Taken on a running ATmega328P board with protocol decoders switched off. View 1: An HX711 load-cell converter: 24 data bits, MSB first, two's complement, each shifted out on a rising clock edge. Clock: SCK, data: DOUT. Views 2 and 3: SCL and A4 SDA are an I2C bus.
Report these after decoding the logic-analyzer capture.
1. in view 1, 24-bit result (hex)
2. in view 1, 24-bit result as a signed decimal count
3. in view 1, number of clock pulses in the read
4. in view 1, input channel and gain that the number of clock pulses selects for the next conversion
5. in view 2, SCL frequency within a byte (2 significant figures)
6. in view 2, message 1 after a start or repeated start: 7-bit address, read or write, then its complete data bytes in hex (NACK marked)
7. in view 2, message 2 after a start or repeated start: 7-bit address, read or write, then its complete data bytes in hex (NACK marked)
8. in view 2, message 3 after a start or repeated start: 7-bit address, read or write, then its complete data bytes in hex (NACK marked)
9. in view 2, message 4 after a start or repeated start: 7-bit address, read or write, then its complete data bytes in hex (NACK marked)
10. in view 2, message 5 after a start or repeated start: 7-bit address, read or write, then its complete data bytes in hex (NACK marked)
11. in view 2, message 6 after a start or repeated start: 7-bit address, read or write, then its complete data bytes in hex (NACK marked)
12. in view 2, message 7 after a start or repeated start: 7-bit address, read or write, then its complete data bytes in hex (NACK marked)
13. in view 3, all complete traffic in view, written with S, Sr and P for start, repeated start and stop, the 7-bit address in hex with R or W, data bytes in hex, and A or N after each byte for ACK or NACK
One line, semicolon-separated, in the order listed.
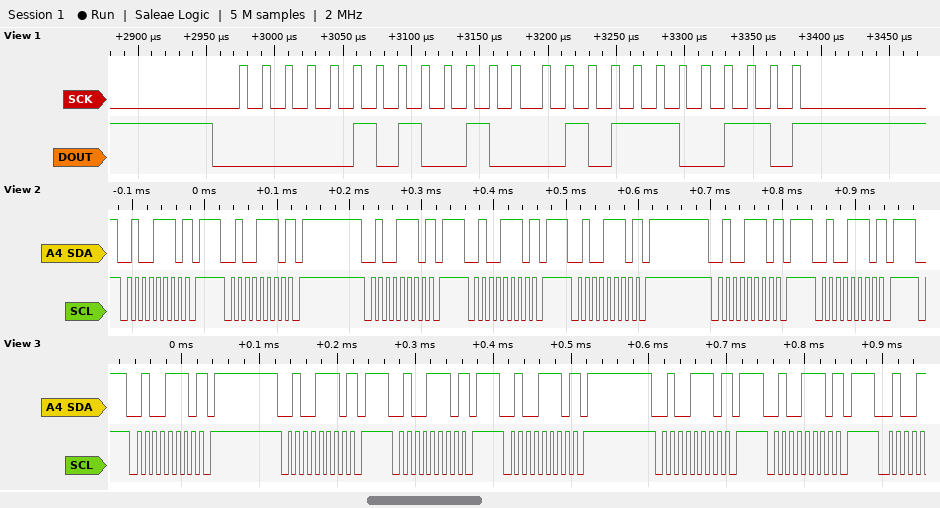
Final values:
0x0522E6; 336614; 25; channel A, gain 128; 100 kHz; 0x27 write NACK; 0x27 write NACK; 0x27 write NACK; 0x27 write NACK; 0x27 write NACK; 0x27 write NACK; 0x27 write NACK; S 27W N P S 27W N P S 27W N P S 27W N P S 27W N P S 27W N P
